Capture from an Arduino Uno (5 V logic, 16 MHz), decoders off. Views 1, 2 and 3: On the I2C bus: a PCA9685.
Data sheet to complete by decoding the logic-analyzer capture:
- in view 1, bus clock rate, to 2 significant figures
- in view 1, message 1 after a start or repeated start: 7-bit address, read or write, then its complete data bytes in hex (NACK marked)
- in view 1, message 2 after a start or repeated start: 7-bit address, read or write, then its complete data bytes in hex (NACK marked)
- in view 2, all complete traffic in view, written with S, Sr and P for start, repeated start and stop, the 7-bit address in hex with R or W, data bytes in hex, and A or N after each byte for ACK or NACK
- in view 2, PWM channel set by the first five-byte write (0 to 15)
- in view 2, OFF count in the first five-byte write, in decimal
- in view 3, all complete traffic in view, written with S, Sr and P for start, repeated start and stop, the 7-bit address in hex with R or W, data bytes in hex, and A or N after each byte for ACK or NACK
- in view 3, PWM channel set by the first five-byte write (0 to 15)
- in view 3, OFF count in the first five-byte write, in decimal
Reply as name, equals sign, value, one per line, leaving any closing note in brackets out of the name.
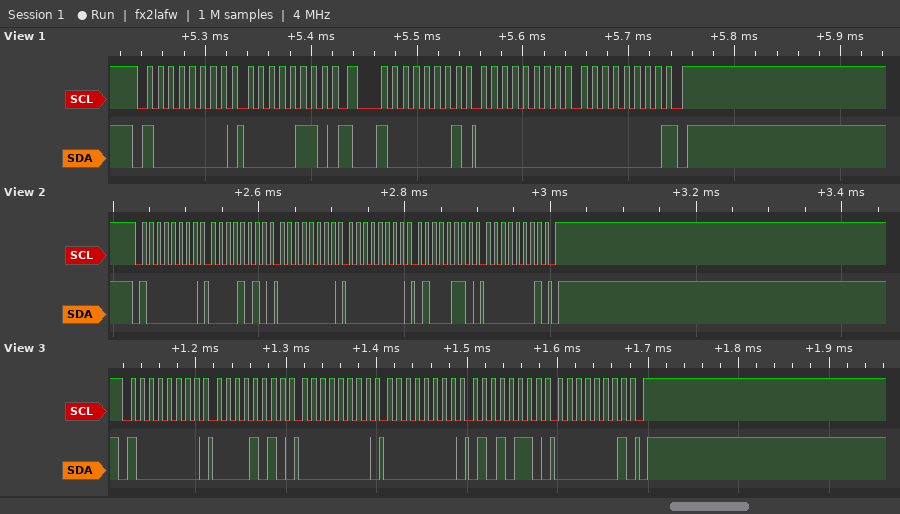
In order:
in view 1, bus clock rate, to 2 significant figures = 100 kHz
in view 1, message 1 after a start or repeated start: 7-bit address, read or write, then its complete data bytes in hex = 0x40 write: 06
in view 1, message 2 after a start or repeated start: 7-bit address, read or write, then its complete data bytes in hex = 0x40 read: 00 00 NACK
in view 2, all complete traffic in view, written with S, Sr and P for start, repeated start and stop, the 7-bit address in hex with R or W, data bytes in hex, and A or N after each byte for ACK or NACK = S 40W A 0A A 00 A 00 A 46 A 01 A P
in view 2, PWM channel set by the first five-byte write = 1
in view 2, OFF count in the first five-byte write, in decimal = 326
in view 3, all complete traffic in view, written with S, Sr and P for start, repeated start and stop, the 7-bit address in hex with R or W, data bytes in hex, and A or N after each byte for ACK or NACK = S 40W A 0A A 00 A 00 A 56 A 01 A P
in view 3, PWM channel set by the first five-byte write = 1
in view 3, OFF count in the first five-byte write, in decimal = 342
